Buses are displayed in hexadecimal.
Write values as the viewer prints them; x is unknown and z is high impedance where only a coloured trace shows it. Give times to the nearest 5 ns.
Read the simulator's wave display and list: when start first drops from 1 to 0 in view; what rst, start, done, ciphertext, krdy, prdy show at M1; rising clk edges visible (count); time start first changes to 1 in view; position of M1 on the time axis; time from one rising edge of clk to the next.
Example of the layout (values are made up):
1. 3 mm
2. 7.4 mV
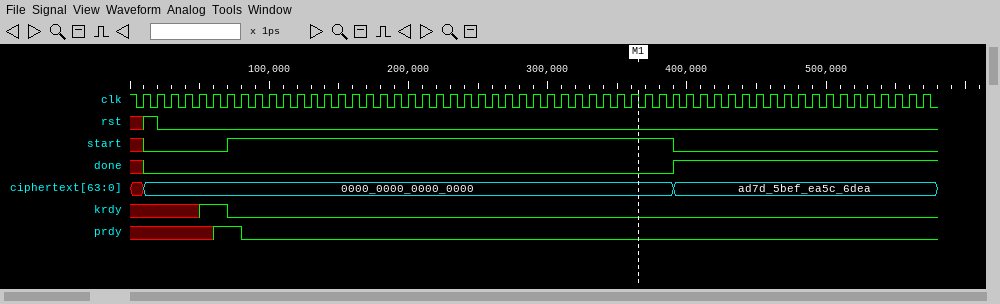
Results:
1. 390 ns
2. rst=0, start=1, done=0, ciphertext=0000_0000_0000_0000, krdy=0, prdy=0
3. 57
4. 70 ns
5. 365 ns
6. 10 ns
